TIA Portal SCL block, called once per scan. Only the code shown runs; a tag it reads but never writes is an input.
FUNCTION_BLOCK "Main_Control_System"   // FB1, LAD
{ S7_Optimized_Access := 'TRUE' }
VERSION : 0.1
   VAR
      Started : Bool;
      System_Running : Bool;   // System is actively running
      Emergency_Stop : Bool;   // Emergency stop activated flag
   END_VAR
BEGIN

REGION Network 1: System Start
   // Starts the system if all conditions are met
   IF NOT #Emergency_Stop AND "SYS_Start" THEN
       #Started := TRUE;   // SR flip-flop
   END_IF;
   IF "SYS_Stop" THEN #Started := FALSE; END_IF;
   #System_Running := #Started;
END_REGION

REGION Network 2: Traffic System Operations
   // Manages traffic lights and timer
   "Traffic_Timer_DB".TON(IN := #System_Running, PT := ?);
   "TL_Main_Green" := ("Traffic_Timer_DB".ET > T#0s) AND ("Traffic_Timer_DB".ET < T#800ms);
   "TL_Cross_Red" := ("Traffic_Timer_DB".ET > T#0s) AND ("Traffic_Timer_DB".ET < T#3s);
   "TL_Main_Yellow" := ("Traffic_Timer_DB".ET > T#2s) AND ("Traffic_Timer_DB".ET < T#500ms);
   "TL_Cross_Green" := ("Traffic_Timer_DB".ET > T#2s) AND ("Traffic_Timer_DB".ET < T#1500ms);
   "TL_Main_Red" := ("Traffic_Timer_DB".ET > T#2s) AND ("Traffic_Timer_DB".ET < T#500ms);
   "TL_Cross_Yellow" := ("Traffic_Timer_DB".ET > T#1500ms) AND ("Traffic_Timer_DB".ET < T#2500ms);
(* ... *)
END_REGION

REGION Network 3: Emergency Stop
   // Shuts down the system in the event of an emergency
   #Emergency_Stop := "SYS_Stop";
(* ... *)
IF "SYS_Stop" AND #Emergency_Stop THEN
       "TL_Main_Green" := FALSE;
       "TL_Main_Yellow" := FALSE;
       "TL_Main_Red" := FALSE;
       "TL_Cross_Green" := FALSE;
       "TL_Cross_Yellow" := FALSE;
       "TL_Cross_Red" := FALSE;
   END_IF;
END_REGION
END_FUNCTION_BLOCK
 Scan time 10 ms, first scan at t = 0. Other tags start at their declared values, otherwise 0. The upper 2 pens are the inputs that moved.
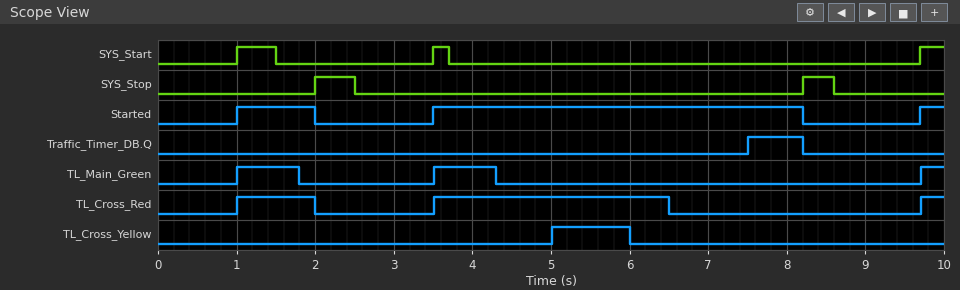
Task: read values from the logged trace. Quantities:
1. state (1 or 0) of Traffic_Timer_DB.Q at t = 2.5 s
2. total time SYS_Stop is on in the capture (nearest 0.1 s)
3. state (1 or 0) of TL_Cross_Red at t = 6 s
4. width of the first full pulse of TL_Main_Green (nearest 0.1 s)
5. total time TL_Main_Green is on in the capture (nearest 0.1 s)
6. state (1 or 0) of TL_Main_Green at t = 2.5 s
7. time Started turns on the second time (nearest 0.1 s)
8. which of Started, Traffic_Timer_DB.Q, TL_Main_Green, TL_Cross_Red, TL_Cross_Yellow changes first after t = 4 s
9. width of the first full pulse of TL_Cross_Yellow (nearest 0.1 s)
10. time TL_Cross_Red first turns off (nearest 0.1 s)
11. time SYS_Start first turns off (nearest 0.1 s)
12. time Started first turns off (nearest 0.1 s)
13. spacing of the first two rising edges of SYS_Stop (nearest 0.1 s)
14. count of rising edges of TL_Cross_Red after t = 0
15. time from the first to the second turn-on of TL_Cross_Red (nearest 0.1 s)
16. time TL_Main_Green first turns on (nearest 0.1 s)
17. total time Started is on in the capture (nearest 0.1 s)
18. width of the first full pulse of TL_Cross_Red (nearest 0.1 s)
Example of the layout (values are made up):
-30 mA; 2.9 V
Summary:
0; 0.9 s; 1; 0.8 s; 1.9 s; 0; 3.5 s; TL_Main_Green; 1.0 s; 2.0 s; 1.5 s; 2.0 s; 6.2 s; 3; 2.5 s; 1.0 s; 6.0 s; 1.0 s
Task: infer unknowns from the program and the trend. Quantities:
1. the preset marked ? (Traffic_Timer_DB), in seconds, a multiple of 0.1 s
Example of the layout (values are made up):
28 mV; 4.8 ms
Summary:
4.0 s
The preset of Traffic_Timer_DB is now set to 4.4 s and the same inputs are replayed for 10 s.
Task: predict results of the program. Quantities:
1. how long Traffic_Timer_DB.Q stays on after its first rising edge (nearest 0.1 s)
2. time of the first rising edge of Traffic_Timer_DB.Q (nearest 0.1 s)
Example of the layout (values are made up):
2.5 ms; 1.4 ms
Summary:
0.3 s; 7.9 s
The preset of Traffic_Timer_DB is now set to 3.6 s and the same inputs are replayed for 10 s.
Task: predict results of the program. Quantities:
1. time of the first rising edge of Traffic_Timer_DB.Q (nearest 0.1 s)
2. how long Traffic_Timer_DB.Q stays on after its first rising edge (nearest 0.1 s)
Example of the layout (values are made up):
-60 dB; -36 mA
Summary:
7.1 s; 1.1 s
